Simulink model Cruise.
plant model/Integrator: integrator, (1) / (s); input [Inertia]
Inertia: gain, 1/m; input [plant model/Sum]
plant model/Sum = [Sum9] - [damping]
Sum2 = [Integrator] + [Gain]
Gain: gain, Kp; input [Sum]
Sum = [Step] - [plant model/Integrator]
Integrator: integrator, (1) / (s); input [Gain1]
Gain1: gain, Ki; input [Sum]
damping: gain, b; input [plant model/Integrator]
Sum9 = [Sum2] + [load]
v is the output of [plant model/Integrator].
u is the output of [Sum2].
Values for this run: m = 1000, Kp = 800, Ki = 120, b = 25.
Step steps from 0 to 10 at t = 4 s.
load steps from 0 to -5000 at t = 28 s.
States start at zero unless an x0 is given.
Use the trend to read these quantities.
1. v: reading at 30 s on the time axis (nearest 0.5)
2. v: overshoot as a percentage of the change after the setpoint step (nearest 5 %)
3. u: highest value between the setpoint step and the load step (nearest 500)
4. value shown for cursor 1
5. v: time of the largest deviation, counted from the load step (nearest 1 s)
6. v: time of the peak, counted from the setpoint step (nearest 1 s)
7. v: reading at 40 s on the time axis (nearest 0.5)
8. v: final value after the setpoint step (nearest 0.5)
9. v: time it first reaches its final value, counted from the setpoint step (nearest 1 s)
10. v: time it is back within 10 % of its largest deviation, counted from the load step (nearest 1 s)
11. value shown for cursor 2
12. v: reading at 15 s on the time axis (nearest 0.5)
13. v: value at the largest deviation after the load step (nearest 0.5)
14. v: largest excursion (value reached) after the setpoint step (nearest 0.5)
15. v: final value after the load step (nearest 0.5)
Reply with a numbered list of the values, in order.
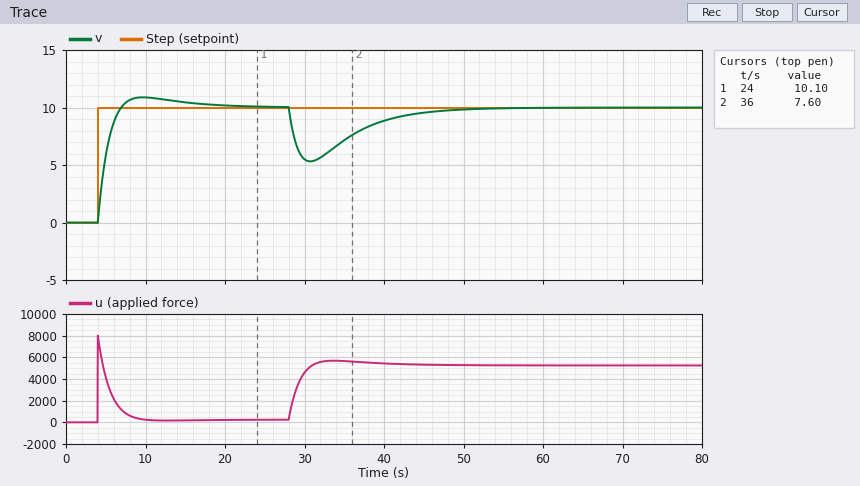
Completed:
1. 5.5
2. 10 %
3. 8000
4. 10.10
5. 3 s
6. 6 s
7. 9.0
8. 10.0
9. 3 s
10. 17 s
11. 7.60
12. 10.5
13. 5.5
14. 11.0
15. 10.0
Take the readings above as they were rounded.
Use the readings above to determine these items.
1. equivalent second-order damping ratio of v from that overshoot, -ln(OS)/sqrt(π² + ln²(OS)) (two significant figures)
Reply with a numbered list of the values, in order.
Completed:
1. 0.59
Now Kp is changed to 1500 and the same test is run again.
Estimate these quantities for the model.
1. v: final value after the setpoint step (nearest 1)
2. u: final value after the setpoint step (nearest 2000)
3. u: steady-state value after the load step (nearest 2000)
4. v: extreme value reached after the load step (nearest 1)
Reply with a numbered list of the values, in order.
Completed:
1. 10
2. 0
3. 6000
4. 7
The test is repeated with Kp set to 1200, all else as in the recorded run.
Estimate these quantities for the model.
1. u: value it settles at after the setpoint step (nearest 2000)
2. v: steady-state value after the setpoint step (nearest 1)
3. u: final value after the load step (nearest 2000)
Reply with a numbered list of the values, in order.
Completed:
1. 0
2. 10
3. 6000
